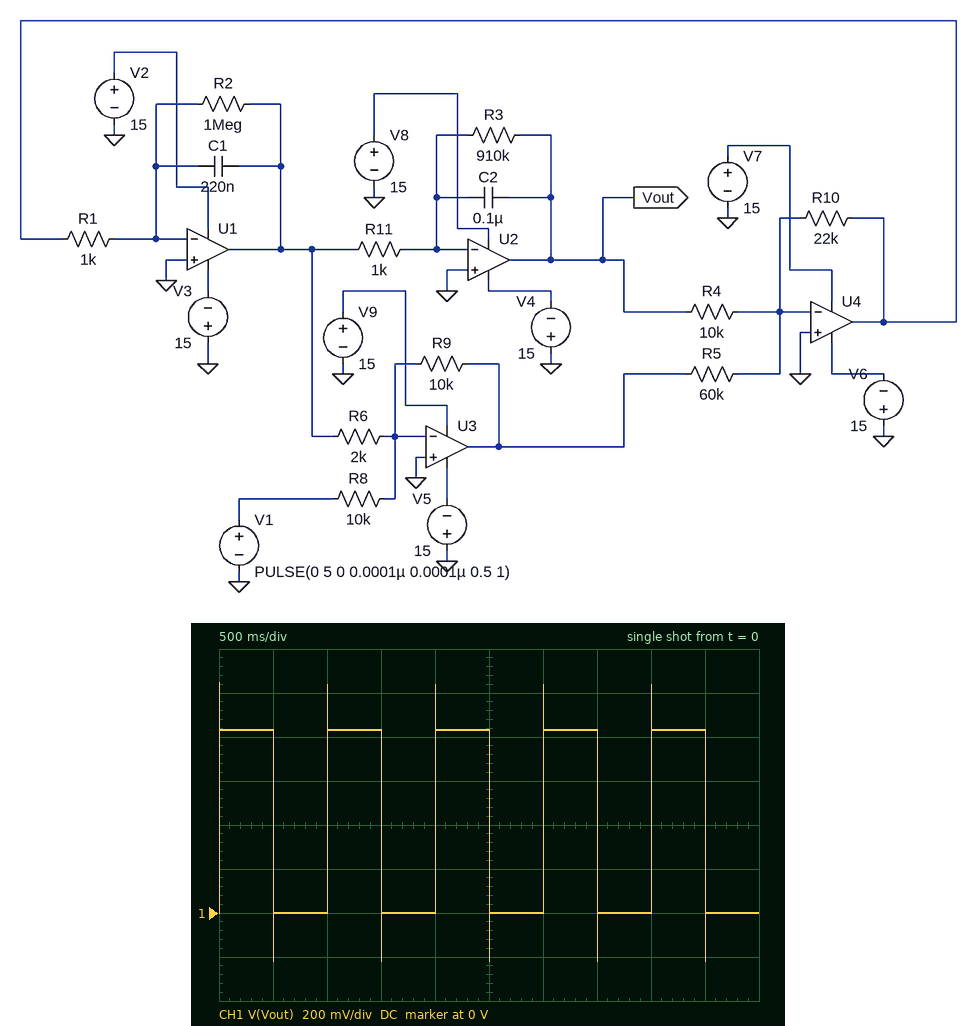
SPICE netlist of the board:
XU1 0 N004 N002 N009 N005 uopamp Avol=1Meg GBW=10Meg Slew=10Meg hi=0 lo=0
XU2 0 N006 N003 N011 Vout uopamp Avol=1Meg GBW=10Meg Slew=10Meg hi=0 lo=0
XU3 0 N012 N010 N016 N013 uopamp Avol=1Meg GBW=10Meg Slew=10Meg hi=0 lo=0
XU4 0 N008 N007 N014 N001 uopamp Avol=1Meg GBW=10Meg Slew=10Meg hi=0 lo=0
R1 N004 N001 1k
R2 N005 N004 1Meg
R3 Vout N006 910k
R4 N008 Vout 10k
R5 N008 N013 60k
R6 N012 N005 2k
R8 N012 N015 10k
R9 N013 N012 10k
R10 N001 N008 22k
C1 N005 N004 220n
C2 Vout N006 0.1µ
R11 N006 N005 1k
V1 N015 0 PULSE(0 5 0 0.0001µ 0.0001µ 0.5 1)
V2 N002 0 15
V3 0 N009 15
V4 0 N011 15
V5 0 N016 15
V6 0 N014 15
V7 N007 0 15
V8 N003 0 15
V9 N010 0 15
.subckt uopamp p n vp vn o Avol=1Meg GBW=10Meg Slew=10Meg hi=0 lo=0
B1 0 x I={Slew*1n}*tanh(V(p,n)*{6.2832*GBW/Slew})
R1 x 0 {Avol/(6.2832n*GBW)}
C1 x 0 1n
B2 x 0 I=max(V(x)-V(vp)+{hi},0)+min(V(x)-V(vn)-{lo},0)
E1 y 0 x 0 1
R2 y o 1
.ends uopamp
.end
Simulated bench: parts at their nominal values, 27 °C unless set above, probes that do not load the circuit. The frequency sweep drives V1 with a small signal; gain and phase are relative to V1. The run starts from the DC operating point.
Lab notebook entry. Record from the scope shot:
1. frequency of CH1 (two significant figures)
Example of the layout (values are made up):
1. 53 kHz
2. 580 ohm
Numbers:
1. 1.0 Hz
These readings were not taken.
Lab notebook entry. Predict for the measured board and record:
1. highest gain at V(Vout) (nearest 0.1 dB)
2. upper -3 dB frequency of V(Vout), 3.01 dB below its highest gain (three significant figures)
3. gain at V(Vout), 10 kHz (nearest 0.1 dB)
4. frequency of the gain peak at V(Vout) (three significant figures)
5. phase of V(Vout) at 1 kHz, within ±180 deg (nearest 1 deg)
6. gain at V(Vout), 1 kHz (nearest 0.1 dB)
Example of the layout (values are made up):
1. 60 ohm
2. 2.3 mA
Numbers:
1. -13.2 dB
2. 1.89 kHz
3. -47.3 dB
4. 1.29 kHz
5. -41 deg
6. -13.6 dB
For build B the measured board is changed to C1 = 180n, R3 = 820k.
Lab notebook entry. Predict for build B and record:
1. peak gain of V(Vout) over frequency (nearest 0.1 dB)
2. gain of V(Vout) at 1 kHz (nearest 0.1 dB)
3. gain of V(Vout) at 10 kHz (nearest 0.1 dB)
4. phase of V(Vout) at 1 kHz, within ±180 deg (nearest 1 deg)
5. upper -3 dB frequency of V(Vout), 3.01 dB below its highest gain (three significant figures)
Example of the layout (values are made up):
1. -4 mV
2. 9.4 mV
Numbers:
1. -13.8 dB
2. -14.2 dB
3. -45.6 dB
4. -38 deg
5. 2.08 kHz
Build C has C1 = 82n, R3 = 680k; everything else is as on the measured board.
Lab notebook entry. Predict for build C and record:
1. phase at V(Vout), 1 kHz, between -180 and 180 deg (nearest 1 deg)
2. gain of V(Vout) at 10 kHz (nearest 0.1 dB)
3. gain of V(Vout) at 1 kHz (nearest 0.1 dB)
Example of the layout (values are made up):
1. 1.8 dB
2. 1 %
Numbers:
1. -32 deg
2. -38.9 dB
3. -15.6 dB
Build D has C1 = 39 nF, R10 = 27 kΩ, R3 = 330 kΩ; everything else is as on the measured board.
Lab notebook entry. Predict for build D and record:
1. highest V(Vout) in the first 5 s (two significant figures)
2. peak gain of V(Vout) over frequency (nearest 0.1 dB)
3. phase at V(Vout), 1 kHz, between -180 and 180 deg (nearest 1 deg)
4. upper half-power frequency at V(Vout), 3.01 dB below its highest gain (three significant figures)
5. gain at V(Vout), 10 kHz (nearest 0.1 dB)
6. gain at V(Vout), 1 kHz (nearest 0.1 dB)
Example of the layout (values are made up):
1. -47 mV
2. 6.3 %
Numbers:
1. 830 mV
2. -15.6 dB
3. -29 deg
4. 2.37 kHz
5. -32.5 dB
6. -16.2 dB
